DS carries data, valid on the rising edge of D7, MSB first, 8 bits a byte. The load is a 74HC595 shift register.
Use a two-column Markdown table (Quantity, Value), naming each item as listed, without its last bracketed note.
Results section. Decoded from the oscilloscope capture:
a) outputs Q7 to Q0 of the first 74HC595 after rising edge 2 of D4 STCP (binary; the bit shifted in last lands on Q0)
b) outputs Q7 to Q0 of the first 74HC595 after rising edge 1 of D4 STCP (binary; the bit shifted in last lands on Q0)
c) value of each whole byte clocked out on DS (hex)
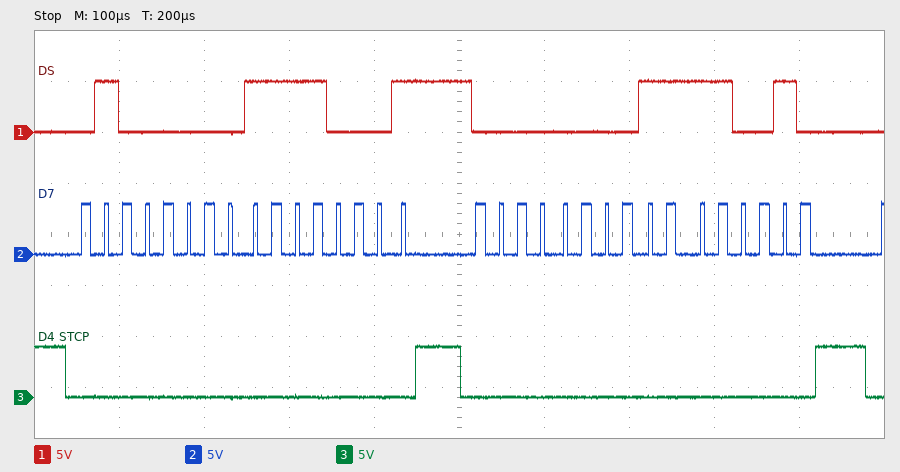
| Quantity | Value |
|---|---|
| outputs Q7 to Q0 of the first 74HC595 after rising edge 2 of D4 STCP | 11110010 |
| outputs Q7 to Q0 of the first 74HC595 after rising edge 1 of D4 STCP | 11110001 |
| value of each whole byte clocked out on DS | 40 F1 00 F2 |
